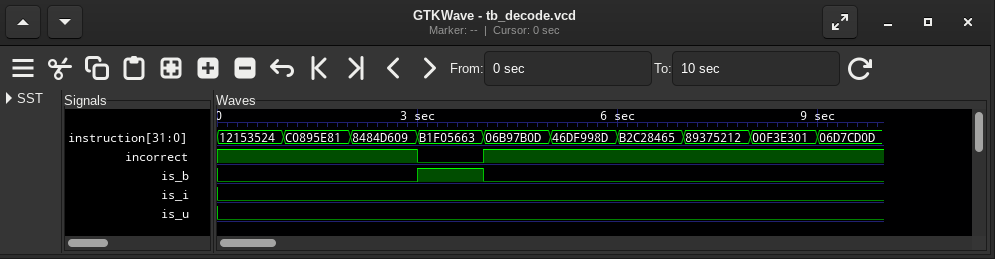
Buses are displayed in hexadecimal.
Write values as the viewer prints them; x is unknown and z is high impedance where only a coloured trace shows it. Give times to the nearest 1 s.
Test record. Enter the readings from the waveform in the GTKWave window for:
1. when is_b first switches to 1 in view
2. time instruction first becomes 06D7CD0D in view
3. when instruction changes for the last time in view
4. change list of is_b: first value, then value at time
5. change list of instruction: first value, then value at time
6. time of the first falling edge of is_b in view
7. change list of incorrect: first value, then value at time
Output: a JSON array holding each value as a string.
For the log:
["3 s", "9 s", "9 s", "0, 1 at 3 s, 0 at 4 s", "12153524, C0895E81 at 1 s, 8484D609 at 2 s, B1F05663 at 3 s, 06B97B0D at 4 s, 46DF998D at 5 s, B2C28465 at 6 s, 89375212 at 7 s, 00F3E301 at 8 s, 06D7CD0D at 9 s", "4 s", "1, 0 at 3 s, 1 at 4 s"]
